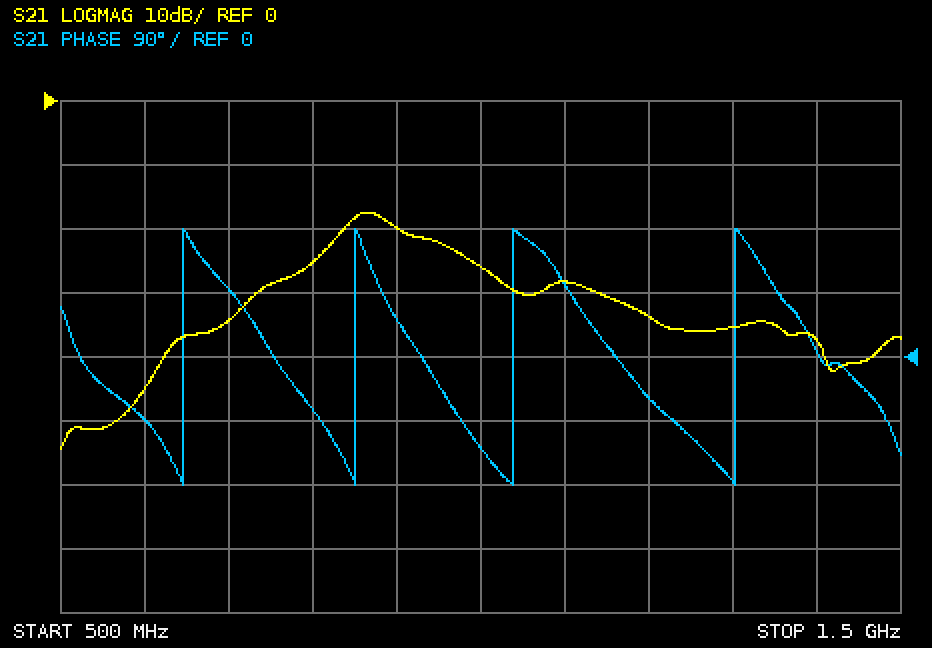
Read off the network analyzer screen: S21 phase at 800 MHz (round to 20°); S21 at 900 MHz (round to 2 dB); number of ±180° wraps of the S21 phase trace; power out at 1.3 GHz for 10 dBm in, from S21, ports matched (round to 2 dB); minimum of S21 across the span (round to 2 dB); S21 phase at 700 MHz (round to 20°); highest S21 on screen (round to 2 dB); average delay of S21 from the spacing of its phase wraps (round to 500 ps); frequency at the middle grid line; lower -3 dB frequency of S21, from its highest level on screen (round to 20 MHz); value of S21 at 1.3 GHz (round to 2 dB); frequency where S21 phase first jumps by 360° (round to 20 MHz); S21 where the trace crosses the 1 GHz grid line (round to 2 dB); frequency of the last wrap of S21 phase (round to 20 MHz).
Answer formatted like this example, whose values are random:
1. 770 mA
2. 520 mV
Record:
1. -80°
2. -20 dB
3. 4
4. -26 dBm
5. -54 dB
6. 100°
7. -18 dB
8. 4.5 ns
9. 1 GHz
10. 840 MHz
11. -36 dB
12. 640 MHz
13. -26 dB
14. 1.30 GHz
